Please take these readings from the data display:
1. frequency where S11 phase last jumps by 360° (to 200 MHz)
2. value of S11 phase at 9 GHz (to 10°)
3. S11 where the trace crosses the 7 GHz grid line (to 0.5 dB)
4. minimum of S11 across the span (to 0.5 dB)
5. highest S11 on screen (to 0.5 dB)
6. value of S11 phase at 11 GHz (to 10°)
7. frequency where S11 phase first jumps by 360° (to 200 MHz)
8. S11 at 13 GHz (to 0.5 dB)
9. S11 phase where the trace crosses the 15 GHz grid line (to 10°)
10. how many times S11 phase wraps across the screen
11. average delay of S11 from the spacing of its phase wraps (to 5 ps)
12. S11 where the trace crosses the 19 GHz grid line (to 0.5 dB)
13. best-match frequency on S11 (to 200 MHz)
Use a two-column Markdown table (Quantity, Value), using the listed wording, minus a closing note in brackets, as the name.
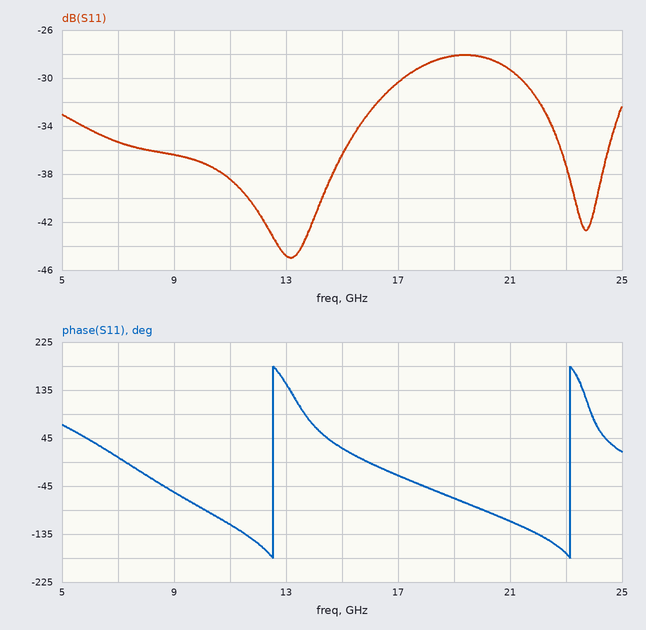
| Quantity | Value |
|---|---|
| frequency where S11 phase last jumps by 360° | 23.2 GHz |
| value of S11 phase at 9 GHz | -60° |
| S11 where the trace crosses the 7 GHz grid line | -35.5 dB |
| minimum of S11 across the span | -45.0 dB |
| highest S11 on screen | -28.0 dB |
| value of S11 phase at 11 GHz | -120° |
| frequency where S11 phase first jumps by 360° | 12.6 GHz |
| S11 at 13 GHz | -45.0 dB |
| S11 phase where the trace crosses the 15 GHz grid line | 30° |
| how many times S11 phase wraps across the screen | 2 |
| average delay of S11 from the spacing of its phase wraps | 95 ps |
| S11 where the trace crosses the 19 GHz grid line | -28.0 dB |
| best-match frequency on S11 | 13.2 GHz |
